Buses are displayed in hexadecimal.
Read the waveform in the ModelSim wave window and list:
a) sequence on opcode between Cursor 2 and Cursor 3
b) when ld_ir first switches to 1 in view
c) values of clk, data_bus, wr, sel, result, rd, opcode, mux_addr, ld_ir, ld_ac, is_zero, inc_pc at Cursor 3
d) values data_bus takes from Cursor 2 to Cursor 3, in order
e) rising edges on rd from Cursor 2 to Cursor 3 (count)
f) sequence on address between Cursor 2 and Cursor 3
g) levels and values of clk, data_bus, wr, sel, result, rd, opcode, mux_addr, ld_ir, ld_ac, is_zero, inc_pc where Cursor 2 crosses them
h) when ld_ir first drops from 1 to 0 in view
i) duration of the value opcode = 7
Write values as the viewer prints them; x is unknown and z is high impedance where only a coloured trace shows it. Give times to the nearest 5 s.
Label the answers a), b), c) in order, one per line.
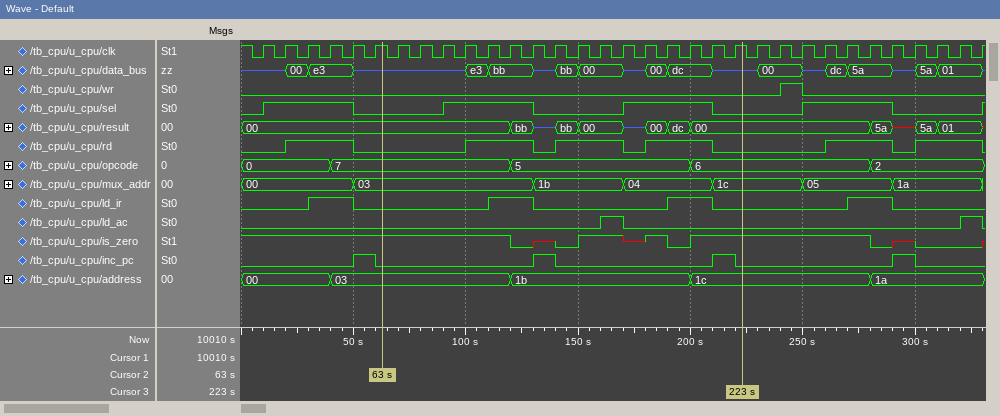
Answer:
a) 7, 5, 6
b) 30 s
c) clk=1, data_bus=z, wr=0, sel=0, result=00, rd=0, opcode=6, mux_addr=1c, ld_ir=0, ld_ac=0, is_zero=1, inc_pc=0
d) z, e3, bb, z, bb, 00, z, 00, dc, z
e) 3
f) 03, 1b, 1c
g) clk=1, data_bus=z, wr=0, sel=0, result=00, rd=0, opcode=7, mux_addr=03, ld_ir=0, ld_ac=0, is_zero=1, inc_pc=0
h) 50 s
i) 80 s
